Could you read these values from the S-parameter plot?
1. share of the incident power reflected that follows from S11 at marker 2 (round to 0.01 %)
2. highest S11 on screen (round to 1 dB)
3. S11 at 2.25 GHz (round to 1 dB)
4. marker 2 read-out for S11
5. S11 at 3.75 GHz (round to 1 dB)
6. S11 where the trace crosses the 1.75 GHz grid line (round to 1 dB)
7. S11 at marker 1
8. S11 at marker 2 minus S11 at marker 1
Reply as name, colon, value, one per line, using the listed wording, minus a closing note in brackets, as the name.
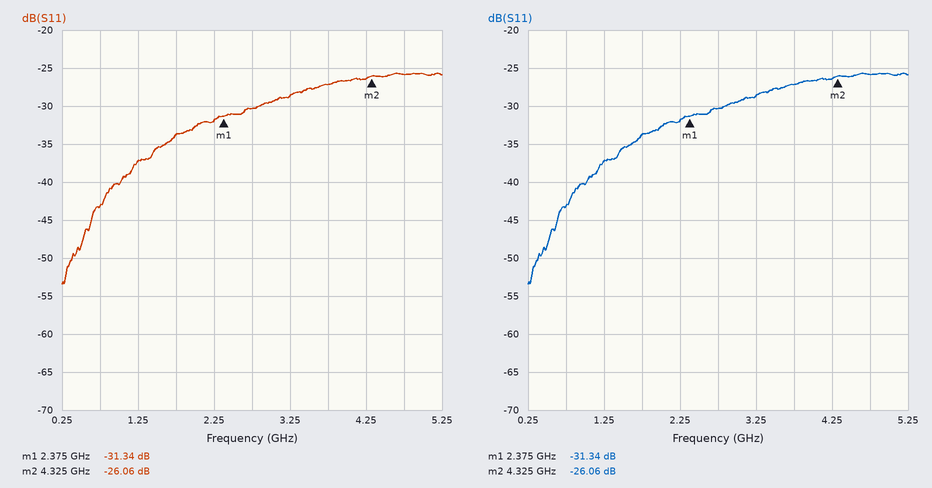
share of the incident power reflected that follows from S11 at marker 2: 0.25 %
highest S11 on screen: -26 dB
S11 at 2.25 GHz: -32 dB
marker 2 read-out for S11: -26.06 dB
S11 at 3.75 GHz: -27 dB
S11 where the trace crosses the 1.75 GHz grid line: -34 dB
S11 at marker 1: -31.34 dB
S11 at marker 2 minus S11 at marker 1: 5.28 dB
